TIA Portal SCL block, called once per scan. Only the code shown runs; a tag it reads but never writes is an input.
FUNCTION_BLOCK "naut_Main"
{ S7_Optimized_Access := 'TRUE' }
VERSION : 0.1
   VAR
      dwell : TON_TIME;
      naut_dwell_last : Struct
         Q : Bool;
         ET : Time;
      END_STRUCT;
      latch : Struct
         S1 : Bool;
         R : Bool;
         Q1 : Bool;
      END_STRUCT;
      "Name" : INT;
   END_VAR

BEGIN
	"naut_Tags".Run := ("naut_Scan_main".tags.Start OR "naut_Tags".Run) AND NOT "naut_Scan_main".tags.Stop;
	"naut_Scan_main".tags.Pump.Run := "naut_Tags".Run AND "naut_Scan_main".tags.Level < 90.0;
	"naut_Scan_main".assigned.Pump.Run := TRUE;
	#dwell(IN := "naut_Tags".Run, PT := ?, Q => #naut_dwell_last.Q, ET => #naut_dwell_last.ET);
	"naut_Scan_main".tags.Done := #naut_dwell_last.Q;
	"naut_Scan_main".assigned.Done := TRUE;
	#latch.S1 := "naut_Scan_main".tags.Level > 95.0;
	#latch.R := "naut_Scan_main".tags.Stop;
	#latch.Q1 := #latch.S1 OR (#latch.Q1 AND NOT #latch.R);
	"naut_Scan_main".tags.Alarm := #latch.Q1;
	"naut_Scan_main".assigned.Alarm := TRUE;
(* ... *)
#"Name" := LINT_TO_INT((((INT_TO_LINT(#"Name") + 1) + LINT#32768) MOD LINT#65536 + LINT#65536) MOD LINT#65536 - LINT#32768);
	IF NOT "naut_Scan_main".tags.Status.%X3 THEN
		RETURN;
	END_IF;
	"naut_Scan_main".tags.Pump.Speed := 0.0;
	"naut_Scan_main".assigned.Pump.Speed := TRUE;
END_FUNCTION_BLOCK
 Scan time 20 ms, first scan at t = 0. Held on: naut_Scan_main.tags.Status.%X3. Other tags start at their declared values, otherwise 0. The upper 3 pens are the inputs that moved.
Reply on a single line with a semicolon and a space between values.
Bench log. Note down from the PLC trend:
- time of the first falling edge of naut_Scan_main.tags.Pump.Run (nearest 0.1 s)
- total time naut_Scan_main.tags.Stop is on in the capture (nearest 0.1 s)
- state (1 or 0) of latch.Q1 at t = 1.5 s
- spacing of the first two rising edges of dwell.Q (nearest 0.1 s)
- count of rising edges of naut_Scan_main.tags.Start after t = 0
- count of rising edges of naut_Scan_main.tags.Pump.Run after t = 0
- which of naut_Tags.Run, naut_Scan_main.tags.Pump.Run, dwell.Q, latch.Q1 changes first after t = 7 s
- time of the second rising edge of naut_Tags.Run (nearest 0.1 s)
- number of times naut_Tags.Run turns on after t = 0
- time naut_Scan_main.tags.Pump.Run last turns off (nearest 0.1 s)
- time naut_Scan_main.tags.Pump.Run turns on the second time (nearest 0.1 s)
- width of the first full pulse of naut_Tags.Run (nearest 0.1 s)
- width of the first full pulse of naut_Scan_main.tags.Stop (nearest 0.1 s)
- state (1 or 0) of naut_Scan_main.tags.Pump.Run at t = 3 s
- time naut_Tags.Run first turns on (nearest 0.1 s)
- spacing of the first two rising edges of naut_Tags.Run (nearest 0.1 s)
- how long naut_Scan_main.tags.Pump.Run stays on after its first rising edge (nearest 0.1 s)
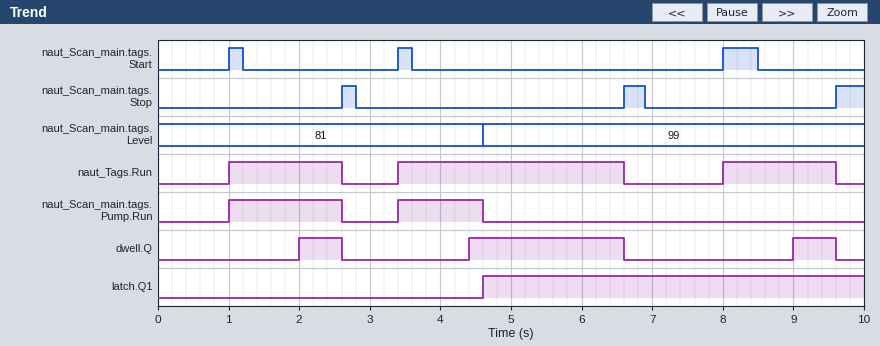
2.6 s; 0.9 s; 0; 2.4 s; 3; 2; naut_Tags.Run; 3.4 s; 3; 4.6 s; 3.4 s; 1.6 s; 0.2 s; 0; 1.0 s; 2.4 s; 1.6 s
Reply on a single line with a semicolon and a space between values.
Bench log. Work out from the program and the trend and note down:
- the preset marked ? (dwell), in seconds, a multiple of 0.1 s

1.0 s
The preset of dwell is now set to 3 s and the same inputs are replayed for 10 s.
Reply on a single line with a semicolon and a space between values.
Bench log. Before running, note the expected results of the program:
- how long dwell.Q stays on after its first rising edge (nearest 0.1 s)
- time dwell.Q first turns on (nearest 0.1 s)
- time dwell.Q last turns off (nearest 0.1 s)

0.2 s; 6.4 s; 6.6 s
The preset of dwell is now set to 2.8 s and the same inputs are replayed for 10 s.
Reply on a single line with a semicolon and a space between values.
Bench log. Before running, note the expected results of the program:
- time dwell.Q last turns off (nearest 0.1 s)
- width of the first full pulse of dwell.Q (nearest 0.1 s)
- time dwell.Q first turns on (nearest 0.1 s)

6.6 s; 0.4 s; 6.2 s
